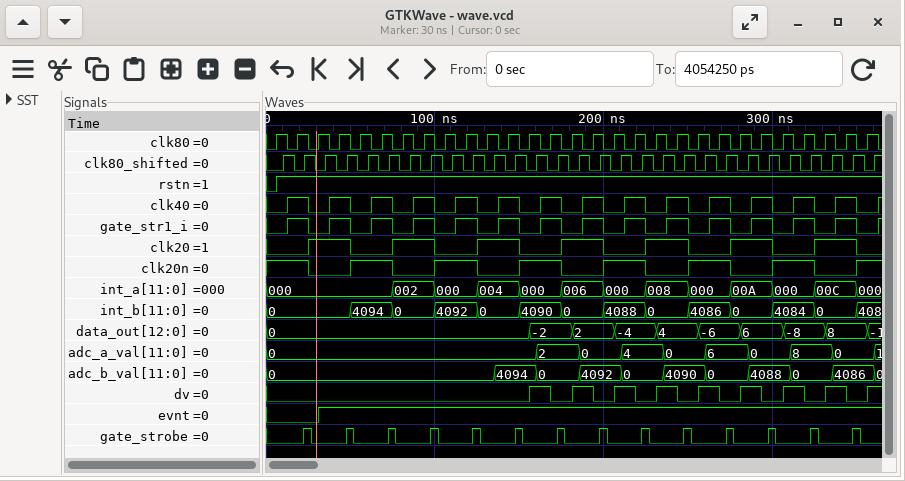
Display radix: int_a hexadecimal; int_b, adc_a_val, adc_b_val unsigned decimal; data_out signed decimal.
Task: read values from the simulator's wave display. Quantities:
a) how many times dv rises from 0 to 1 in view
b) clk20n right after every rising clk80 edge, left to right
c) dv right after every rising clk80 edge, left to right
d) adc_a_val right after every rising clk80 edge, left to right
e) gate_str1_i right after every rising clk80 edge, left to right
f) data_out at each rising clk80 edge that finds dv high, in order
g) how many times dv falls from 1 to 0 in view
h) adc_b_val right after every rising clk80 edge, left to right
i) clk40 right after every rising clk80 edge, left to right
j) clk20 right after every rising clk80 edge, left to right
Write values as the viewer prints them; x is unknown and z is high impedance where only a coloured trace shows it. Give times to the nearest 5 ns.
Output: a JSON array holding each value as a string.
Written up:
["9", "1 1 0 0 1 1 0 0 1 1 0 0 1 1 0 0 1 1 0 0 1 1 0 0 1 1 0 0 1", "0 0 0 0 0 0 0 0 0 0 0 0 1 0 1 0 1 0 1 0 1 0 1 0 1 0 1 0 1", "0, 0, 0, 0, 0, 0, 0, 0, 0, 0, 0, 0, 0, 2, 2, 0, 0, 4, 4, 0, 0, 6, 6, 0, 0, 8, 8, 0, 0", "0 1 0 1 0 1 0 1 0 1 0 1 0 1 0 1 0 1 0 1 0 1 0 1 0 1 0 1 0", "-2, 2, -4, 4, -6, 6, -8, 8", "8", "0, 0, 0, 0, 0, 0, 0, 0, 0, 0, 0, 4094, 4094, 0, 0, 4092, 4092, 0, 0, 4090, 4090, 0, 0, 4088, 4088, 0, 0, 4086, 4086", "0 1 0 1 0 1 0 1 0 1 0 1 0 1 0 1 0 1 0 1 0 1 0 1 0 1 0 1 0", "0 0 1 1 0 0 1 1 0 0 1 1 0 0 1 1 0 0 1 1 0 0 1 1 0 0 1 1 0"]
